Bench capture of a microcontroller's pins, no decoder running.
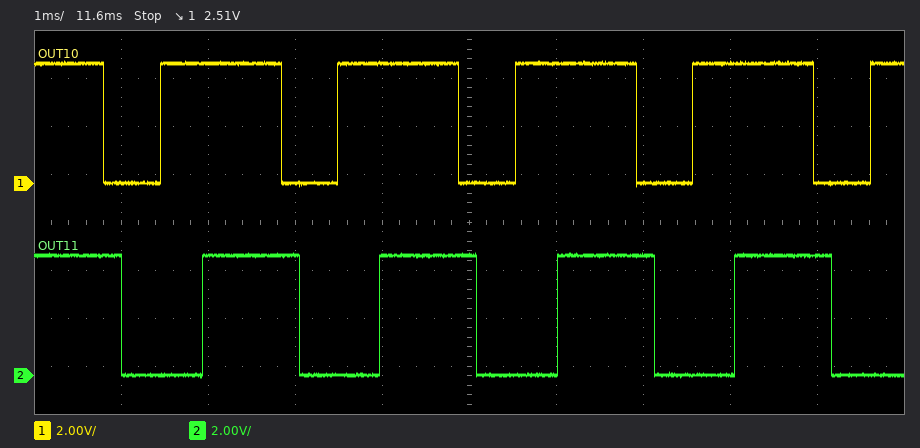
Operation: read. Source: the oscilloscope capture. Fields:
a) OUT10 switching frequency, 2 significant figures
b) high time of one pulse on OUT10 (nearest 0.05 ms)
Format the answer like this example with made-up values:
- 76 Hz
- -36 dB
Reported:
- 490 Hz
- 1.40 ms
